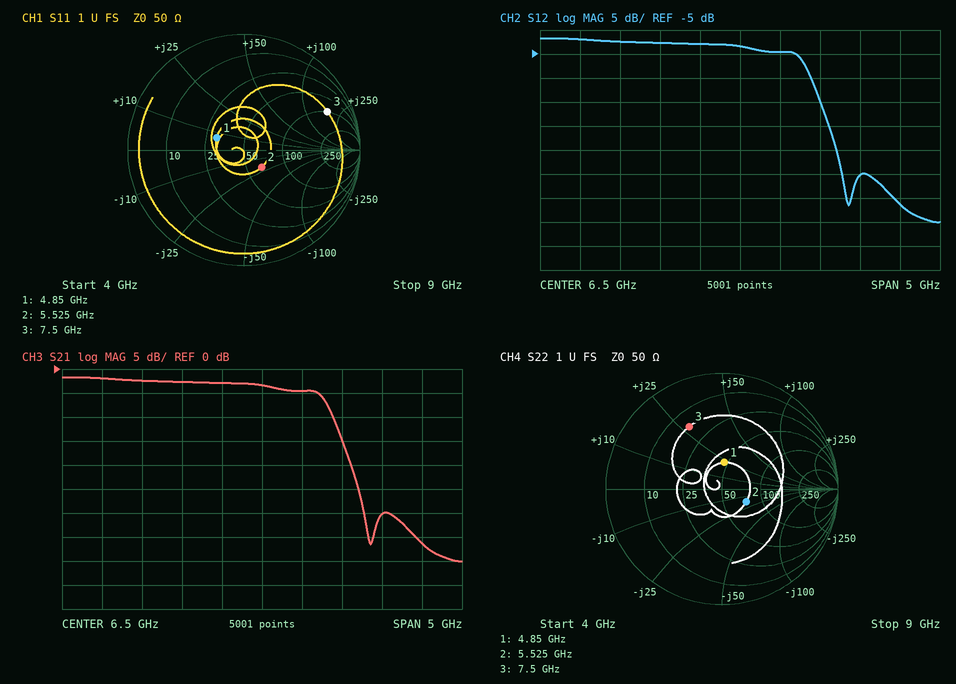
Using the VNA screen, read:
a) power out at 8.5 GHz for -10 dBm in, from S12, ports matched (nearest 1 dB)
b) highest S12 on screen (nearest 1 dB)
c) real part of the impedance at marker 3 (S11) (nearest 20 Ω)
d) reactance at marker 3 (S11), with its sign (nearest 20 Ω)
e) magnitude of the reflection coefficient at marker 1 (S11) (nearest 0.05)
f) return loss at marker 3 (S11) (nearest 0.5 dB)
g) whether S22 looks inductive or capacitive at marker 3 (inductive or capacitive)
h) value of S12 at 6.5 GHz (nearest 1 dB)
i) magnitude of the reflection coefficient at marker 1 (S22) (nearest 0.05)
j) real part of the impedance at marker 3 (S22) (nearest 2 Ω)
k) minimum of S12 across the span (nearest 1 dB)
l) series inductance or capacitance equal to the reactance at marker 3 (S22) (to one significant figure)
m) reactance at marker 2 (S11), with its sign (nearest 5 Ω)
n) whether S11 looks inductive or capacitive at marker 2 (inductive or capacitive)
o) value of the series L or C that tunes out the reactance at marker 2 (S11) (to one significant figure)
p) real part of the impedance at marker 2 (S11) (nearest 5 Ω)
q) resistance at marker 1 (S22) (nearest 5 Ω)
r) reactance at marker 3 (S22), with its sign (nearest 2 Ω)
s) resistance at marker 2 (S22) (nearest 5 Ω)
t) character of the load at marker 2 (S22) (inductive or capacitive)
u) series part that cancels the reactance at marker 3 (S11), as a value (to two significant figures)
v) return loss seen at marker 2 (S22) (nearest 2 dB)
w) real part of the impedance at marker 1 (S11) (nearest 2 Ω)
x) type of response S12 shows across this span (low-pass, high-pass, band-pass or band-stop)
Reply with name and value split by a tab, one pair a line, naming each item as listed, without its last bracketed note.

power out at 8.5 GHz for -10 dBm in, from S12, ports matched	-46 dBm
highest S12 on screen	-2 dB
real part of the impedance at marker 3 (S11)	100 Ω
reactance at marker 3 (S11), with its sign	+180 Ω
magnitude of the reflection coefficient at marker 1 (S11)	0.25
return loss at marker 3 (S11)	2.0 dB
whether S22 looks inductive or capacitive at marker 3	inductive
value of S12 at 6.5 GHz	-3 dB
magnitude of the reflection coefficient at marker 1 (S22)	0.25
real part of the impedance at marker 3 (S22)	16 Ω
minimum of S12 across the span	-40 dB
series inductance or capacitance equal to the reactance at marker 3 (S22)	600 pH
reactance at marker 2 (S11), with its sign	-20 Ω
whether S11 looks inductive or capacitive at marker 2	capacitive
value of the series L or C that tunes out the reactance at marker 2 (S11)	600 pH
real part of the impedance at marker 2 (S11)	65 Ω
resistance at marker 1 (S22)	45 Ω
reactance at marker 3 (S22), with its sign	+28 Ω
resistance at marker 2 (S22)	75 Ω
character of the load at marker 2 (S22)	capacitive
series part that cancels the reactance at marker 3 (S11), as a value	120 fF
return loss seen at marker 2 (S22)	12 dB
real part of the impedance at marker 1 (S11)	30 Ω
type of response S12 shows across this span	low-pass
